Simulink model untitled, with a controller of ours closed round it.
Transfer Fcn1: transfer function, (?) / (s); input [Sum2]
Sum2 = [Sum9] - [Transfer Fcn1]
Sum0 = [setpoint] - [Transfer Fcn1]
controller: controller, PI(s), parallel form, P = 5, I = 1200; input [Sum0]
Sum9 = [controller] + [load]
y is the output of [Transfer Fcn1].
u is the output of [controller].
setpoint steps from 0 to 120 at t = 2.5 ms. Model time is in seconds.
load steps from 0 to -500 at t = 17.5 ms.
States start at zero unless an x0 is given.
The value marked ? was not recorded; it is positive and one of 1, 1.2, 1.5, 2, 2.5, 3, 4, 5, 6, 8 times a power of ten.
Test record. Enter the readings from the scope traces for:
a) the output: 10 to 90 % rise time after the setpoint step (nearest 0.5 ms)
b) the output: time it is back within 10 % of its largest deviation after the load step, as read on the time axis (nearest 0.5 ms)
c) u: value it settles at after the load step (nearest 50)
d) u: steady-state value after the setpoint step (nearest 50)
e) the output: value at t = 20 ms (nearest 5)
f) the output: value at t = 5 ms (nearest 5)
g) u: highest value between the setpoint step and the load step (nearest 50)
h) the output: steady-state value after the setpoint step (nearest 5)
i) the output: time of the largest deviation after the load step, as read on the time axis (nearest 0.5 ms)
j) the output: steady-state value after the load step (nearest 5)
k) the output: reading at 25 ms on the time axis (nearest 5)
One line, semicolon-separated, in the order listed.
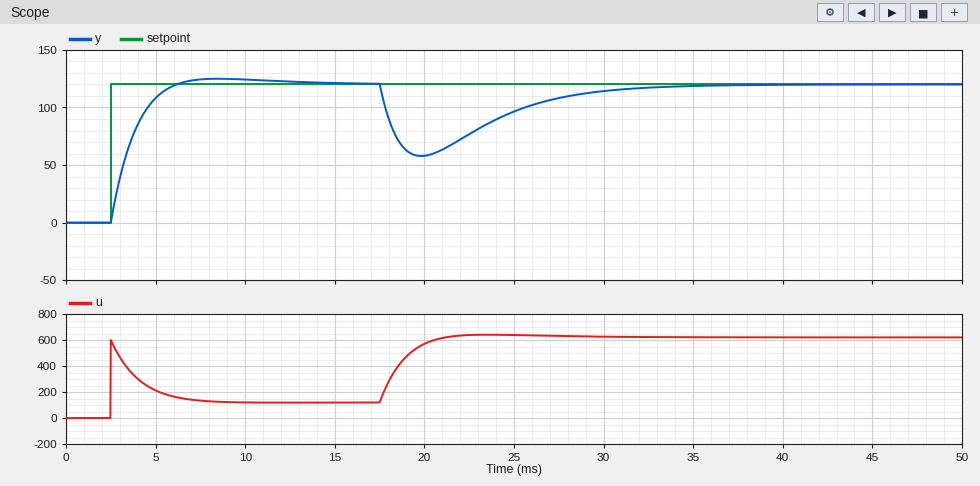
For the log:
2.5 ms; 29.5 ms; 600; 100; 60; 110; 600; 120; 20.0 ms; 120; 95
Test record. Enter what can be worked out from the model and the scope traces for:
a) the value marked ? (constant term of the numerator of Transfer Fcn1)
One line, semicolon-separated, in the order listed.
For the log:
150
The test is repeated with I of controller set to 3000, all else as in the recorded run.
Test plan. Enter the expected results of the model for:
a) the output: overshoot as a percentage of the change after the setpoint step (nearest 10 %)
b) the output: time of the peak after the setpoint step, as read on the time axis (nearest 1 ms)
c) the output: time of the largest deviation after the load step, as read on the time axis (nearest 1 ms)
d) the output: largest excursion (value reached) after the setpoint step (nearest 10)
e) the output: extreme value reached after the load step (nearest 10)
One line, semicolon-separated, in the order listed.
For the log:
20 %; 6 ms; 19 ms; 140; 70
